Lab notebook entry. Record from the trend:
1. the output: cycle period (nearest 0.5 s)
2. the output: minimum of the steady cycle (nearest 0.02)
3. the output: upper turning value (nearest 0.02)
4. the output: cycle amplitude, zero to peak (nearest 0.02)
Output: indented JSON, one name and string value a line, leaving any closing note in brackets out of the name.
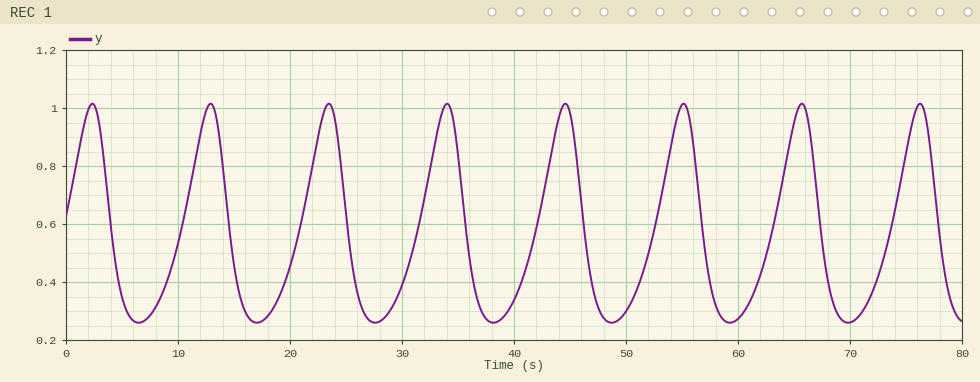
{
  "the output: cycle period": "10.5 s",
  "the output: minimum of the steady cycle": "0.26",
  "the output: upper turning value": "1.02",
  "the output: cycle amplitude, zero to peak": "0.38"
}
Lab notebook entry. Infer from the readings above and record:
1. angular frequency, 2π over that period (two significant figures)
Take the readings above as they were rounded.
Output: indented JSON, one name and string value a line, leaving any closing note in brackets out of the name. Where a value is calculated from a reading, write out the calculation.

{
  "angular frequency, 2π over that period": "2π / 10.5 = 0.60 rad/s"
}
